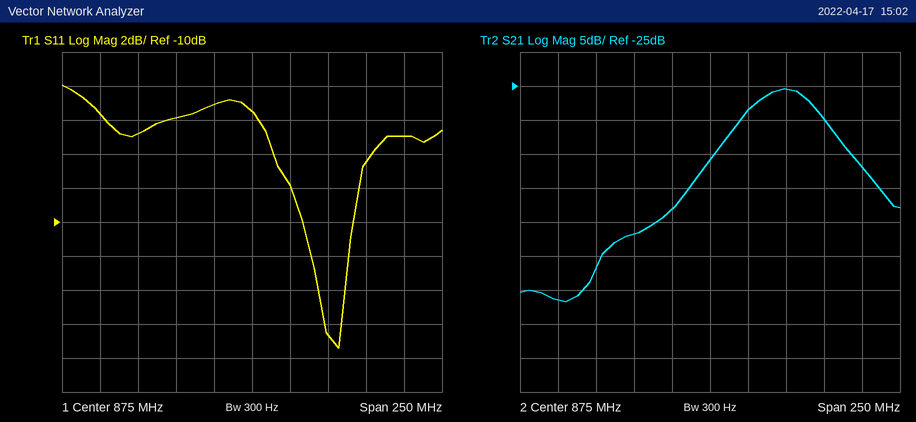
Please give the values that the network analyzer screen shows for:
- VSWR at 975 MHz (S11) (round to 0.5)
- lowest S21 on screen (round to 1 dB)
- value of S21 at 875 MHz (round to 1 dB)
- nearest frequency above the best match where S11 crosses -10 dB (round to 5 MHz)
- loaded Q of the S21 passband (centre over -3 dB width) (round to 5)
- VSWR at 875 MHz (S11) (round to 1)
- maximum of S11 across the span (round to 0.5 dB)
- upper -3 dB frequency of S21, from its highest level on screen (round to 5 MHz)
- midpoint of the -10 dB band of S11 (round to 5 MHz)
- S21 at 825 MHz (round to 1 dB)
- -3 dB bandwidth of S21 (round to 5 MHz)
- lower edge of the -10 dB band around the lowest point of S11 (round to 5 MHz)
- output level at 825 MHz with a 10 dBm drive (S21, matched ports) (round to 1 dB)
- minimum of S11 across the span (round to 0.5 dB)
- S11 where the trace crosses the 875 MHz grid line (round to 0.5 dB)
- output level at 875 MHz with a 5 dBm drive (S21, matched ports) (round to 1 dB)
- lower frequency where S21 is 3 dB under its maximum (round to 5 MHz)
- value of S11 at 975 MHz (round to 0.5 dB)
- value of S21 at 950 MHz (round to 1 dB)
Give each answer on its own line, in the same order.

3.5
-57 dB
-36 dB
940 MHz
20
5
-2.0 dB
945 MHz
925 MHz
-47 dB
45 MHz
910 MHz
-37 dBm
-17.5 dB
-3.5 dB
-31 dBm
900 MHz
-5.0 dB
-30 dB
